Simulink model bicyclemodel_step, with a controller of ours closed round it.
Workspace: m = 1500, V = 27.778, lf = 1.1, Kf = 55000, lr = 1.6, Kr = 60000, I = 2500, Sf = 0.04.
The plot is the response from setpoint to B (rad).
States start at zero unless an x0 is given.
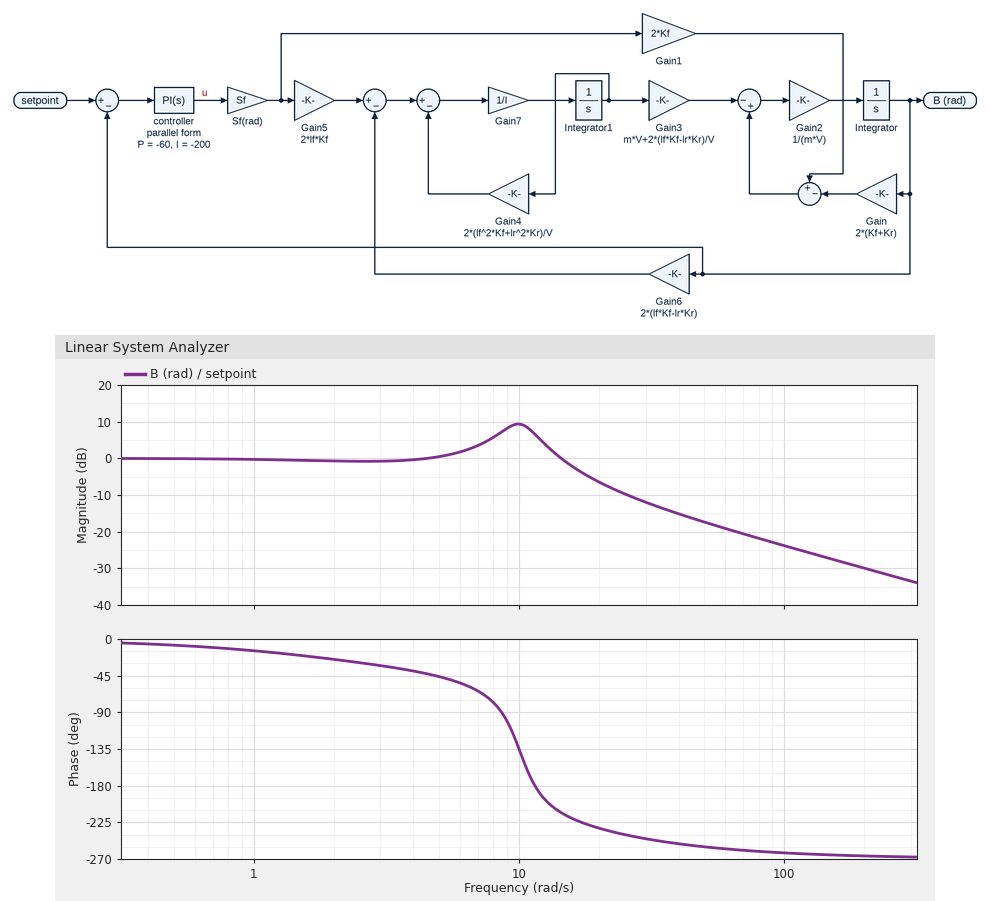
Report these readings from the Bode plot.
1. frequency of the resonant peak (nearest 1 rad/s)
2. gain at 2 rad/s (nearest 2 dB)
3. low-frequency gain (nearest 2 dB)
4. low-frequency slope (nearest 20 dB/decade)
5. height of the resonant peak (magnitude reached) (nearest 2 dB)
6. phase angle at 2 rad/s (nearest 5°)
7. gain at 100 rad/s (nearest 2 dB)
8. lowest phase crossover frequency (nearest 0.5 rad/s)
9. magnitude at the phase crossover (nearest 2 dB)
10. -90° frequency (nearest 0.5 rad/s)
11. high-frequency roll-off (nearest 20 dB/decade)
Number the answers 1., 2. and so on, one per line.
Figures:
1. 10 rad/s
2. 0 dB
3. 0 dB
4. 0 dB/decade
5. 10 dB
6. -25°
7. -24 dB
8. 11.5 rad/s
9. 6 dB
10. 8.5 rad/s
11. -20 dB/decade
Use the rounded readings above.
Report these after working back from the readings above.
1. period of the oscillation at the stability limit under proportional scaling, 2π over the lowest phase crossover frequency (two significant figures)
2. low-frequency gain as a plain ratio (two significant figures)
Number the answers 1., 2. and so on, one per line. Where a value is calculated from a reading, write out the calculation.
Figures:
1. 2π / 11.5 = 0.55 s
2. 10^(0 / 20) = 1.0
